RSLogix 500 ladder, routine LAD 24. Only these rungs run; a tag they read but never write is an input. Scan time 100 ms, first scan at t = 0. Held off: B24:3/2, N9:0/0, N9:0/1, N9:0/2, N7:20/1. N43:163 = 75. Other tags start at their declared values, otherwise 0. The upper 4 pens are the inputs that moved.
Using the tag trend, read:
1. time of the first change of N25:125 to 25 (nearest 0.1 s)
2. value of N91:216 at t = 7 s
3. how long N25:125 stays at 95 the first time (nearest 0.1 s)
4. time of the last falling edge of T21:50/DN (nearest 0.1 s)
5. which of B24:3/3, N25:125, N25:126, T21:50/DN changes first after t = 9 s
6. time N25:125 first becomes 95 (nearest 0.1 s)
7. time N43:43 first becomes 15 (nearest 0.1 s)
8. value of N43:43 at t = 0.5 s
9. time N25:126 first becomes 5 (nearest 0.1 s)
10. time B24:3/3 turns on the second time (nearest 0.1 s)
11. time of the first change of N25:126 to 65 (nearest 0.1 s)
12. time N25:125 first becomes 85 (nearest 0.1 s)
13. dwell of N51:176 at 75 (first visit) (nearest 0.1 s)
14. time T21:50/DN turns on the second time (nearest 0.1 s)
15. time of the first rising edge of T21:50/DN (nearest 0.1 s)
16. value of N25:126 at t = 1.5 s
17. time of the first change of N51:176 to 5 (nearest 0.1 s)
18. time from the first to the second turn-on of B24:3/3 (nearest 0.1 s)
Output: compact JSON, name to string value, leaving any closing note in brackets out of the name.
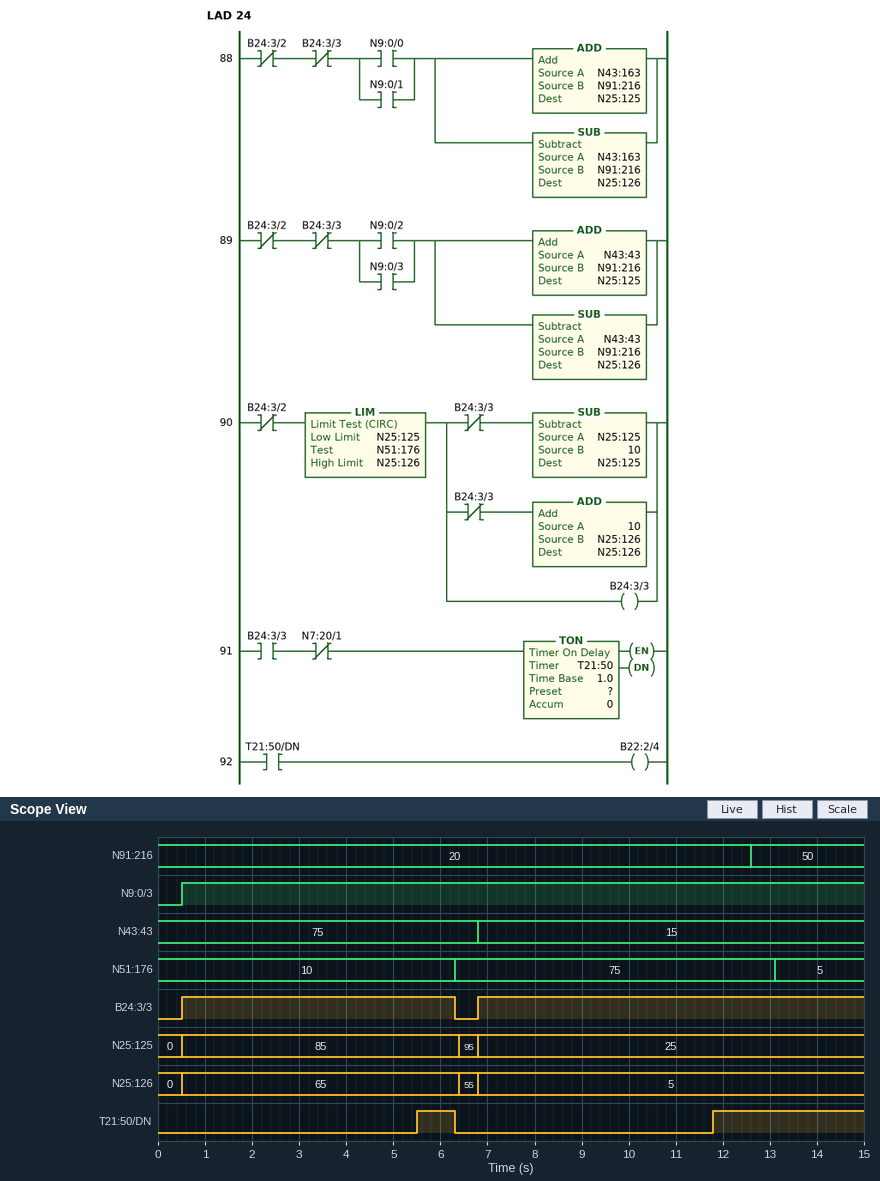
{"time of the first change of N25:125 to 25": "6.8 s", "value of N91:216 at t = 7 s": "20", "how long N25:125 stays at 95 the first time": "0.4 s", "time of the last falling edge of T21:50/DN": "6.3 s", "which of B24:3/3, N25:125, N25:126, T21:50/DN changes first after t = 9 s": "T21:50/DN", "time N25:125 first becomes 95": "6.4 s", "time N43:43 first becomes 15": "6.8 s", "value of N43:43 at t = 0.5 s": "75", "time N25:126 first becomes 5": "6.8 s", "time B24:3/3 turns on the second time": "6.8 s", "time of the first change of N25:126 to 65": "0.5 s", "time N25:125 first becomes 85": "0.5 s", "dwell of N51:176 at 75 (first visit)": "6.8 s", "time T21:50/DN turns on the second time": "11.8 s", "time of the first rising edge of T21:50/DN": "5.5 s", "value of N25:126 at t = 1.5 s": "65", "time of the first change of N51:176 to 5": "13.1 s", "time from the first to the second turn-on of B24:3/3": "6.3 s"}
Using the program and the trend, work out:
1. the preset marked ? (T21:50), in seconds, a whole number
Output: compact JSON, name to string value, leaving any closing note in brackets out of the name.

{"the preset marked ? (T21:50), in seconds, a whole number": "5 s"}
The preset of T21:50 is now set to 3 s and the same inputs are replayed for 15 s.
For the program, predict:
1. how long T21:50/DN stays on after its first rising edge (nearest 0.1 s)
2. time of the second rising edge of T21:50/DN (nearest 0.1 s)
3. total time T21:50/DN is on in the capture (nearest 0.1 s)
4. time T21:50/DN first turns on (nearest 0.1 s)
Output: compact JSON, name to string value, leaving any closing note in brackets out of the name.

{"how long T21:50/DN stays on after its first rising edge": "2.8 s", "time of the second rising edge of T21:50/DN": "9.8 s", "total time T21:50/DN is on in the capture": "8.0 s", "time T21:50/DN first turns on": "3.5 s"}
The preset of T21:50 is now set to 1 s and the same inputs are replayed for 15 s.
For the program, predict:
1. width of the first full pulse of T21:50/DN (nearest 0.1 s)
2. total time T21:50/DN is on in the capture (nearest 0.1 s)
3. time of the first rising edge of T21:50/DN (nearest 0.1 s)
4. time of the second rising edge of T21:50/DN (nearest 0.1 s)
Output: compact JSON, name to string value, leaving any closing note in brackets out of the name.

{"width of the first full pulse of T21:50/DN": "4.8 s", "total time T21:50/DN is on in the capture": "12.0 s", "time of the first rising edge of T21:50/DN": "1.5 s", "time of the second rising edge of T21:50/DN": "7.8 s"}
